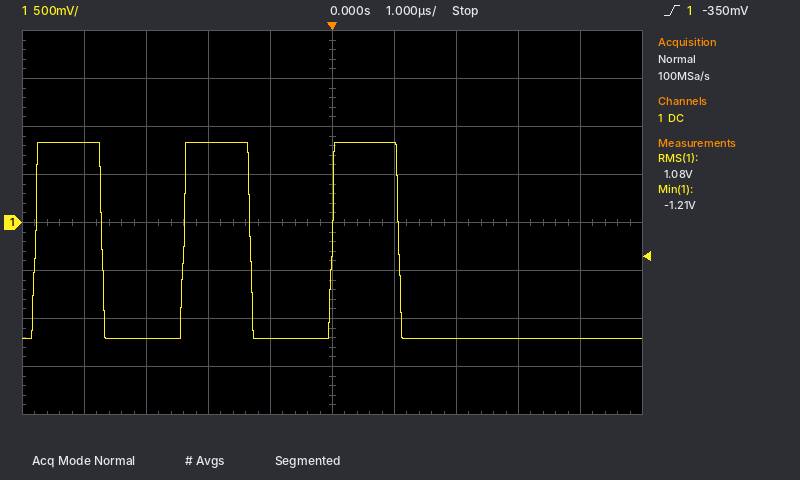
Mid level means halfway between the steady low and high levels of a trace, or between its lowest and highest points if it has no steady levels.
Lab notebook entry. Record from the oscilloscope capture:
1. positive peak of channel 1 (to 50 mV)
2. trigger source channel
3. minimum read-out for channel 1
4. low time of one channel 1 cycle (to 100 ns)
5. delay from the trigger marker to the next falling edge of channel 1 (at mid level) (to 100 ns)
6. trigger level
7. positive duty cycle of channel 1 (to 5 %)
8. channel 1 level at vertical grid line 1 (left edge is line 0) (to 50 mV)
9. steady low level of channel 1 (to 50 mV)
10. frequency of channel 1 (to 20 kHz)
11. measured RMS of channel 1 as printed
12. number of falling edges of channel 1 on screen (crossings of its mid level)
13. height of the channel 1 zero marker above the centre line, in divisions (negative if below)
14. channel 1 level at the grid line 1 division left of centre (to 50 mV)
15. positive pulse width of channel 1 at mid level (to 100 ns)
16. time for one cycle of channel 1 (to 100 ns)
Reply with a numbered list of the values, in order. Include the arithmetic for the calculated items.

1. 850 mV
2. channel 1
3. -1.21 V
4. 1.3 µs
5. 1.1 µs
6. -350 mV
7. 1.1 µs / 2.4 µs ≈ 45.8 %, so 45 % to the nearest 5 %
8. 850 mV
9. -1.20 V
10. 1 / 2.4 µs ≈ 417 kHz, so 420 kHz to the nearest 20 kHz
11. 1.08 V
12. 3
13. 0.0 div
14. -1.20 V
15. 1.1 µs
16. 2.4 µs
